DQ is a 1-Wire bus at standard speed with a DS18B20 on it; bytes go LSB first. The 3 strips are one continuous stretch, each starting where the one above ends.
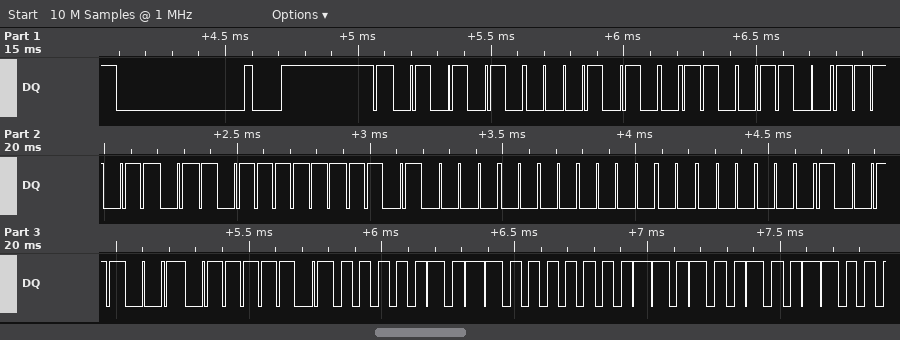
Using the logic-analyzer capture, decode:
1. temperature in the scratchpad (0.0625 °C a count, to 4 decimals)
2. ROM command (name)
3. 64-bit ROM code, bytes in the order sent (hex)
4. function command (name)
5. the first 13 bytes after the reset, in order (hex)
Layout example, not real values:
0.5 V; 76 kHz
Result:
26.0000 °C; Match ROM; 28 33 B7 FD 0B 00 00 99; Read Scratchpad; 55 28 33 B7 FD 0B 00 00 99 BE A0 01 4B
